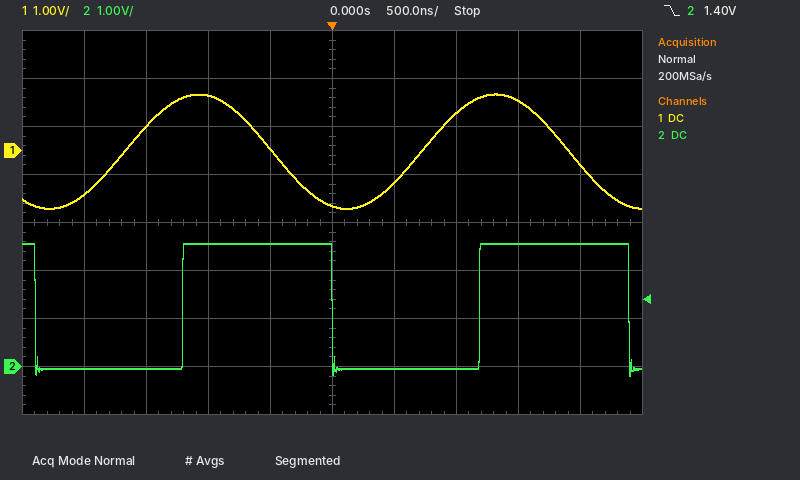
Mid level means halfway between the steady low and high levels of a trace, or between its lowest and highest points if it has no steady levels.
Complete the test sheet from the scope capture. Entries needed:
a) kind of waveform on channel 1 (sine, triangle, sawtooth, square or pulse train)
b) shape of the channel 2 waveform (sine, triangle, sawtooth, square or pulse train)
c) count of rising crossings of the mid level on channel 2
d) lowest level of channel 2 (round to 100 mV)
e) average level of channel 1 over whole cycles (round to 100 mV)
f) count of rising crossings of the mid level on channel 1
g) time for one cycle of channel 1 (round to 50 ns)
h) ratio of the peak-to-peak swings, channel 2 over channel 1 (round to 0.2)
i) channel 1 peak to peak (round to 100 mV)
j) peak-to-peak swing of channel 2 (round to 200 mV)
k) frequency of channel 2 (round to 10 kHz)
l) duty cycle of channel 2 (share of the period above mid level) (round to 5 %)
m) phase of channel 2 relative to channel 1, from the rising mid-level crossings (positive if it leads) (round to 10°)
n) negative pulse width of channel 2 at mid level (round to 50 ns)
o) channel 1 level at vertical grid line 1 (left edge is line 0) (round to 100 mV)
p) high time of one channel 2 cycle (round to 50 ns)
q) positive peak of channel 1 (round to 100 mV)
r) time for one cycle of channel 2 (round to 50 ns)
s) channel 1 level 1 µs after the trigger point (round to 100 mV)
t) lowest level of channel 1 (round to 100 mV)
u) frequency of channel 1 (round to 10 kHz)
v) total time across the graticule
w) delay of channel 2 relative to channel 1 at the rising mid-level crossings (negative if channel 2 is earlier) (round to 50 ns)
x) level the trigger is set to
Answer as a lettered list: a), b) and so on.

a) sine
b) square
c) 2
d) -200 mV
e) 0.0 V
f) 2
g) 2.40 µs
h) 1.2
i) 2.4 V
j) 2.8 V
k) 420 kHz
l) 50 %
m) -70°
n) 1.20 µs
o) -900 mV
p) 1.20 µs
q) 1.2 V
r) 2.40 µs
s) 800 mV
t) -1.2 V
u) 420 kHz
v) 5 µs
w) +450 ns
x) 1.40 V
